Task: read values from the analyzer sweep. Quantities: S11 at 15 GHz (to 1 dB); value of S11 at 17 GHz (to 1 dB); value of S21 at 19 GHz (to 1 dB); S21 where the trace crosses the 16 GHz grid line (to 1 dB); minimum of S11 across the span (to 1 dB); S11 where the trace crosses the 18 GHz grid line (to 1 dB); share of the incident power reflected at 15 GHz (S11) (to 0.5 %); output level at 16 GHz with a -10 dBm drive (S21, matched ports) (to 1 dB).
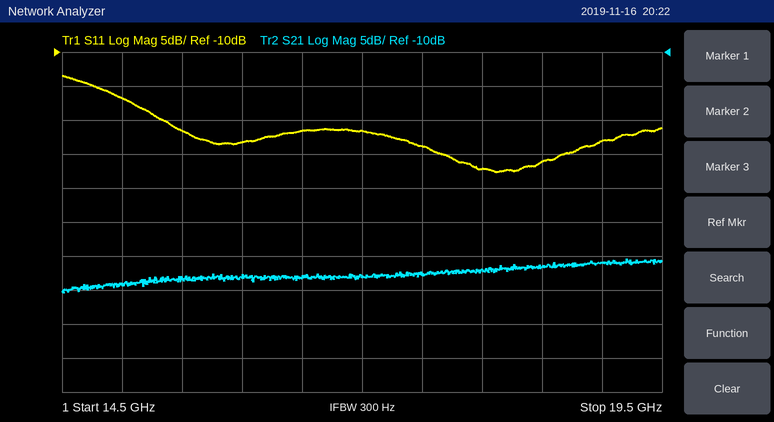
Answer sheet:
-17 dB
-22 dB
-41 dB
-43 dB
-28 dB
-27 dB
2.0 %
-53 dBm
